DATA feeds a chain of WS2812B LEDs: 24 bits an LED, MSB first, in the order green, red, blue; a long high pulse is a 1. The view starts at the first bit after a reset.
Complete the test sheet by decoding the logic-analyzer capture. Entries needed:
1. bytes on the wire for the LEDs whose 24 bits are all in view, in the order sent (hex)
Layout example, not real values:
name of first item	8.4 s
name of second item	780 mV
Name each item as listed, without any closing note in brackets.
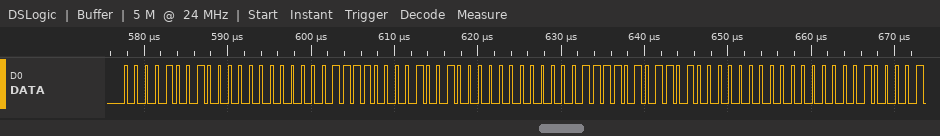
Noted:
bytes on the wire for the LEDs whose 24 bits are all in view, in the order sent	09 00 0F 09 00 0F 5A 00 01
